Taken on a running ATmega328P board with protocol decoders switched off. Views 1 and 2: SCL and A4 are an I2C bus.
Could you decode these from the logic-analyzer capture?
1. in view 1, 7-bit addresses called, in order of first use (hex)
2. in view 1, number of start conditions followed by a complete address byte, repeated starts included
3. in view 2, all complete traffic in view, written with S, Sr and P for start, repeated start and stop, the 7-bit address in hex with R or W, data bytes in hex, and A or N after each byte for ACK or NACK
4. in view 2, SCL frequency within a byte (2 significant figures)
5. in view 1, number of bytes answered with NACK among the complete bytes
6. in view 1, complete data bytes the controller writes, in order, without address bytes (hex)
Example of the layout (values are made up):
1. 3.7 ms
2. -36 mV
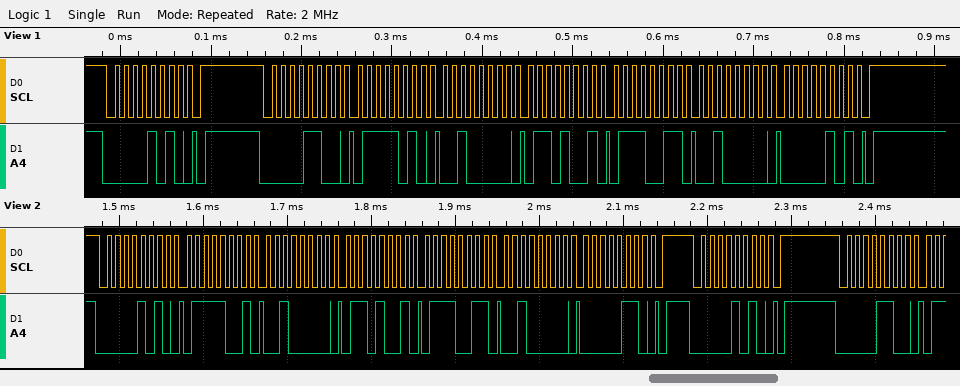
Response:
1. 0x05 0x06
2. 2
3. S 05W A 79 A 20 A 69 A 73 A 20 A 06 A P S 05W A P S 06W A
4. 100 kHz
5. 0
6. 7A 20 69 73 20 05
